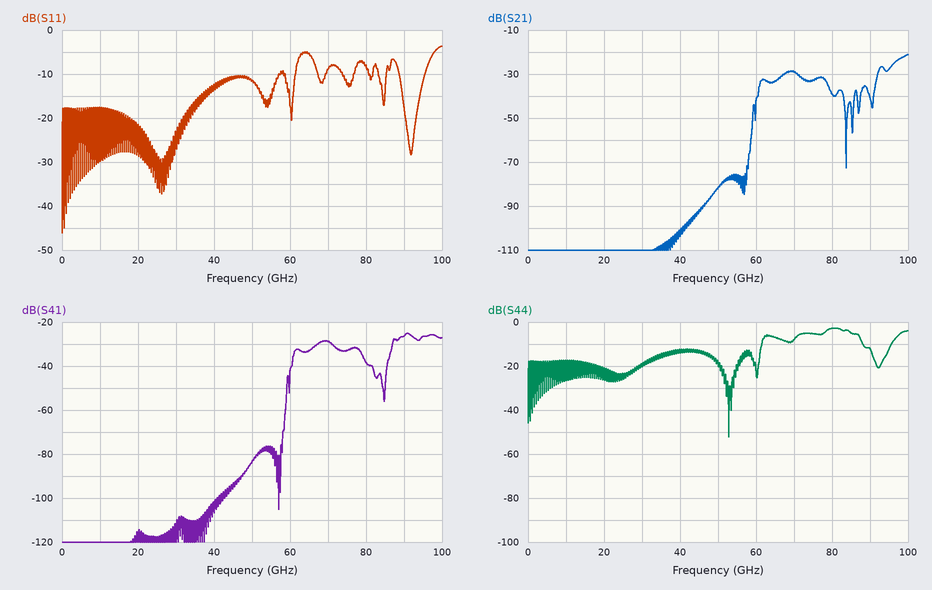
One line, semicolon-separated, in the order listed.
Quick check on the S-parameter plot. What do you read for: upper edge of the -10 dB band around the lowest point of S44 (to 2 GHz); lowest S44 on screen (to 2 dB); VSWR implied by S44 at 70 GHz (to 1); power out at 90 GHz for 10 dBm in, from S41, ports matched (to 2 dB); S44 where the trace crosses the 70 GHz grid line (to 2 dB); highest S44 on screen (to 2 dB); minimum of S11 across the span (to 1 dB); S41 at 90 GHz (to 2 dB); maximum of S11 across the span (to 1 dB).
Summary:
62 GHz; -52 dB; 2; -16 dBm; -8 dB; -2 dB; -46 dB; -26 dB; -4 dB
